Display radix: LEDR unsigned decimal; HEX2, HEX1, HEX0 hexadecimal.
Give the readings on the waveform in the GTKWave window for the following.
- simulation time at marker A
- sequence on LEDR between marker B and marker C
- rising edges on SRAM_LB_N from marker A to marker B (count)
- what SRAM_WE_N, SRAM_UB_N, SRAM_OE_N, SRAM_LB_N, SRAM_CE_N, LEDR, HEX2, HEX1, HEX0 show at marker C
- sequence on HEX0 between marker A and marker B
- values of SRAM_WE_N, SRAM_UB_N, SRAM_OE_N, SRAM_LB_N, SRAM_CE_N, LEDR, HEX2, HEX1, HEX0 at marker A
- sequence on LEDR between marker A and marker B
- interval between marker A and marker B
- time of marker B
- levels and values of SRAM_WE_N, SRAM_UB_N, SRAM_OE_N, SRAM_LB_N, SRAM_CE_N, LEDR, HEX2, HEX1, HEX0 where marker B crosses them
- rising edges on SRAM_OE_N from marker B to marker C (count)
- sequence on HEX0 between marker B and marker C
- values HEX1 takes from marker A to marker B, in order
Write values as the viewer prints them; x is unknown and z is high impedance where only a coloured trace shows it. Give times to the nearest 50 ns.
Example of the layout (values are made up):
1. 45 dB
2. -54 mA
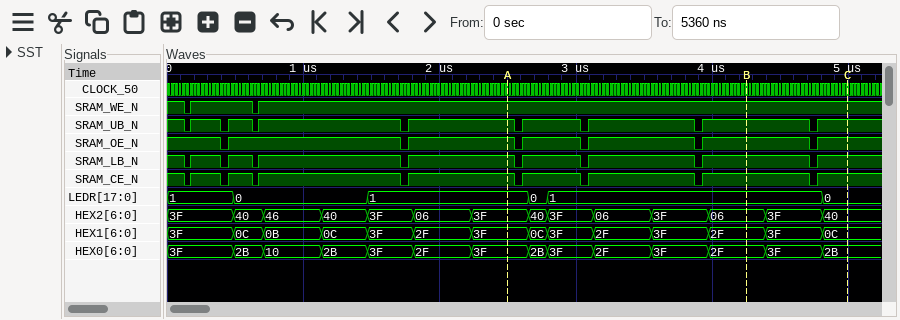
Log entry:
1. 2500 ns
2. 1, 0
3. 3
4. SRAM_WE_N=1, SRAM_UB_N=1, SRAM_OE_N=1, SRAM_LB_N=1, SRAM_CE_N=1, LEDR=0, HEX2=40, HEX1=0C, HEX0=2B
5. 3F, 2B, 3F, 2F, 3F, 2F
6. SRAM_WE_N=1, SRAM_UB_N=1, SRAM_OE_N=1, SRAM_LB_N=1, SRAM_CE_N=1, LEDR=1, HEX2=3F, HEX1=3F, HEX0=3F
7. 1, 0, 1
8. 1750 ns
9. 4250 ns
10. SRAM_WE_N=1, SRAM_UB_N=1, SRAM_OE_N=1, SRAM_LB_N=1, SRAM_CE_N=1, LEDR=1, HEX2=06, HEX1=2F, HEX0=2F
11. 1
12. 2F, 3F, 2B
13. 3F, 0C, 3F, 2F, 3F, 2F
